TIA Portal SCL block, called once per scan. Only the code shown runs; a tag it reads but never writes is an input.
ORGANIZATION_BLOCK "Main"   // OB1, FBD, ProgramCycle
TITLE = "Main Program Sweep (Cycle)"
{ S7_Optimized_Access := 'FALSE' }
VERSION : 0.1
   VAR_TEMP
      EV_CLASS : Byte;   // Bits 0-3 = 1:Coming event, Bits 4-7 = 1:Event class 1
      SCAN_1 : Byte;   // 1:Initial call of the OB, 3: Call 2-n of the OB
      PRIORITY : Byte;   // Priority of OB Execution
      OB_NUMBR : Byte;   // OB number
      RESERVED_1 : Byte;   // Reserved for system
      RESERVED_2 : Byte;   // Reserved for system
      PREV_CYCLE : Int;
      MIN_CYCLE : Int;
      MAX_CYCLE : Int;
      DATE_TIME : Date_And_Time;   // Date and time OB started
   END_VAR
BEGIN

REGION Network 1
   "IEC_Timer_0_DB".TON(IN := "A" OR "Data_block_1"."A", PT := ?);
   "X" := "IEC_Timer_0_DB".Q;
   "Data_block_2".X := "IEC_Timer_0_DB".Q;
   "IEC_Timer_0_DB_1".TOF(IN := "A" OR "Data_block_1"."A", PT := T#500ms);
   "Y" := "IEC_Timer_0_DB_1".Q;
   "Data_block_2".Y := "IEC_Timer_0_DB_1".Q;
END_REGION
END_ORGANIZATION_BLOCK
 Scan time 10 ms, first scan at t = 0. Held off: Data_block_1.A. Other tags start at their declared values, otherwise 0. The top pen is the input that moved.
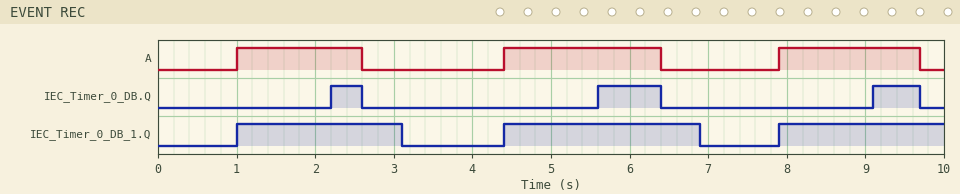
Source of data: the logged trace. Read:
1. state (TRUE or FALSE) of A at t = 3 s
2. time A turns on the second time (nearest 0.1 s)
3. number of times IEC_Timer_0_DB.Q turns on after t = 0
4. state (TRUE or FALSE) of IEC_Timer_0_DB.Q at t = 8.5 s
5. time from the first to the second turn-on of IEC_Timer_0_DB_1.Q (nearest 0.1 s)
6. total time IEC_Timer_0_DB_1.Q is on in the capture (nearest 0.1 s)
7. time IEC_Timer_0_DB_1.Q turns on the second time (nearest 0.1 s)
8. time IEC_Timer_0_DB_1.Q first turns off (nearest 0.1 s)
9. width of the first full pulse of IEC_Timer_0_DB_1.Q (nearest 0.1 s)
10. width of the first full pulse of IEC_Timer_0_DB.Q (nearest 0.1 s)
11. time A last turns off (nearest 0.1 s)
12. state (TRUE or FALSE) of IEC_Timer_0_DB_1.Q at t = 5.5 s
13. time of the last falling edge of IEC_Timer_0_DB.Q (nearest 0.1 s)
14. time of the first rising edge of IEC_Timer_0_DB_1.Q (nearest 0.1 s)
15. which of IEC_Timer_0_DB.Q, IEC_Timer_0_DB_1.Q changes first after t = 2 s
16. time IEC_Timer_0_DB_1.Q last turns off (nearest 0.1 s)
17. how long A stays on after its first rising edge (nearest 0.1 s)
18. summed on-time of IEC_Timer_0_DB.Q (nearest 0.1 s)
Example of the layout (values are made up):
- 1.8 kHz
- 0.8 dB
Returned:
- FALSE
- 4.4 s
- 3
- FALSE
- 3.4 s
- 6.7 s
- 4.4 s
- 3.1 s
- 2.1 s
- 0.4 s
- 9.7 s
- TRUE
- 9.7 s
- 1.0 s
- IEC_Timer_0_DB.Q
- 6.9 s
- 1.6 s
- 1.8 s
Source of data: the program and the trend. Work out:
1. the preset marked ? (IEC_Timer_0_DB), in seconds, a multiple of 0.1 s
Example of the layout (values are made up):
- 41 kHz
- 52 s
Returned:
- 1.2 s
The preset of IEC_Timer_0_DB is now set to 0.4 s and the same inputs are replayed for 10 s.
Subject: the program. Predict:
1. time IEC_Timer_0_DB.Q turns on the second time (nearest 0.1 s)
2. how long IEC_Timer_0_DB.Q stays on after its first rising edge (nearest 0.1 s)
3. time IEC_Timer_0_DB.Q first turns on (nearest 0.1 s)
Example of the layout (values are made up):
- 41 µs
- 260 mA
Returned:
- 4.8 s
- 1.2 s
- 1.4 s
